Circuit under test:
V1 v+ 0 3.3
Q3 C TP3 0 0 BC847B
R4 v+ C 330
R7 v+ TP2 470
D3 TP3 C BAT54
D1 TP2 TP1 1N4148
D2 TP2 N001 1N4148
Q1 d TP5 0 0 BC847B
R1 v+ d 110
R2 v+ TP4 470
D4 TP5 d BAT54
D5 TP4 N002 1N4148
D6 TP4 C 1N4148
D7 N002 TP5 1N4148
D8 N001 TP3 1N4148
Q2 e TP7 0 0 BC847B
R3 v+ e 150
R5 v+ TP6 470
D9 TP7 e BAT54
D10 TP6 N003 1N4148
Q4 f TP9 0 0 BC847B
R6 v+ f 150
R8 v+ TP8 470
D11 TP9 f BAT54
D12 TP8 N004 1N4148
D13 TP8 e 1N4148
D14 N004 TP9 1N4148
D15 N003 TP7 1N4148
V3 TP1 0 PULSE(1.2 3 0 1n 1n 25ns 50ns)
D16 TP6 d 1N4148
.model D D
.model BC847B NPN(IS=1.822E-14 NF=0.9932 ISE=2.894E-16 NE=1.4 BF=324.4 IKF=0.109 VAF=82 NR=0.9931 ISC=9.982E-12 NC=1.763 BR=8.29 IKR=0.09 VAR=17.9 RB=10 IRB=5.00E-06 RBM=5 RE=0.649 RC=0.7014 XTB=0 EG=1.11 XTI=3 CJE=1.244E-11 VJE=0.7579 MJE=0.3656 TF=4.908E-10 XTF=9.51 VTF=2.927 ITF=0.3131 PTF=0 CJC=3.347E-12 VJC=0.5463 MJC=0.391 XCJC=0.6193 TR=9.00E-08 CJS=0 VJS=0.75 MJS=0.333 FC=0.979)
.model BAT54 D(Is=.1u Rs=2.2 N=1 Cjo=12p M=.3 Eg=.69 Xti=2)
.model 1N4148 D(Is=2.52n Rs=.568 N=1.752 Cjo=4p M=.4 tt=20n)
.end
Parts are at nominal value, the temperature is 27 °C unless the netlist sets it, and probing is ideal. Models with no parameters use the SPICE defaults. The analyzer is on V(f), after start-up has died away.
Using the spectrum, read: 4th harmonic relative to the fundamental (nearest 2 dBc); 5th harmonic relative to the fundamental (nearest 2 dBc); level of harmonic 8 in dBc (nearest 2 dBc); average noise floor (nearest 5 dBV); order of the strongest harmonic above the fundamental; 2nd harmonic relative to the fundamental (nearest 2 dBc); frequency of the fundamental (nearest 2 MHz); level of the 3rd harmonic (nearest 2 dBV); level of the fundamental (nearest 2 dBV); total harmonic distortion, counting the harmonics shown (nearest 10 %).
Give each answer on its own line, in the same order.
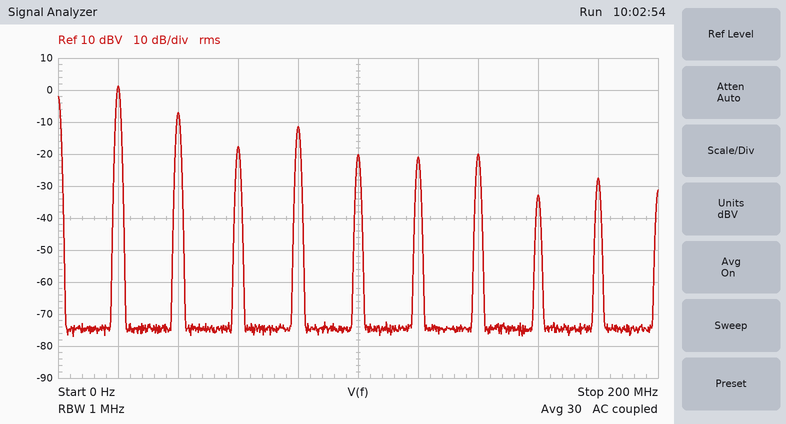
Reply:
-12 dBc
-22 dBc
-34 dBc
-75 dBV
2
-8 dBc
20 MHz
-18 dBV
2 dBV
50 %
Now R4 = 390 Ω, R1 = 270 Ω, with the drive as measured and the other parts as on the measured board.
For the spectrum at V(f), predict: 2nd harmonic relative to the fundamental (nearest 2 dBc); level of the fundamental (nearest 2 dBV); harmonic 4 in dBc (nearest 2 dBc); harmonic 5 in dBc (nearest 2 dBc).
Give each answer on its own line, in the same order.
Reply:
-12 dBc
2 dBV
-14 dBc
-26 dBc
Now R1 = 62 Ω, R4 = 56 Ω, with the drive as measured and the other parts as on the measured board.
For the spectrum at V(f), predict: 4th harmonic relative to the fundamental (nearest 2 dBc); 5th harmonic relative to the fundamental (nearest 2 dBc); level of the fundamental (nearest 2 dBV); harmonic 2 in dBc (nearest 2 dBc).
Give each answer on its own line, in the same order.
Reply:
-14 dBc
-28 dBc
2 dBV
-12 dBc
